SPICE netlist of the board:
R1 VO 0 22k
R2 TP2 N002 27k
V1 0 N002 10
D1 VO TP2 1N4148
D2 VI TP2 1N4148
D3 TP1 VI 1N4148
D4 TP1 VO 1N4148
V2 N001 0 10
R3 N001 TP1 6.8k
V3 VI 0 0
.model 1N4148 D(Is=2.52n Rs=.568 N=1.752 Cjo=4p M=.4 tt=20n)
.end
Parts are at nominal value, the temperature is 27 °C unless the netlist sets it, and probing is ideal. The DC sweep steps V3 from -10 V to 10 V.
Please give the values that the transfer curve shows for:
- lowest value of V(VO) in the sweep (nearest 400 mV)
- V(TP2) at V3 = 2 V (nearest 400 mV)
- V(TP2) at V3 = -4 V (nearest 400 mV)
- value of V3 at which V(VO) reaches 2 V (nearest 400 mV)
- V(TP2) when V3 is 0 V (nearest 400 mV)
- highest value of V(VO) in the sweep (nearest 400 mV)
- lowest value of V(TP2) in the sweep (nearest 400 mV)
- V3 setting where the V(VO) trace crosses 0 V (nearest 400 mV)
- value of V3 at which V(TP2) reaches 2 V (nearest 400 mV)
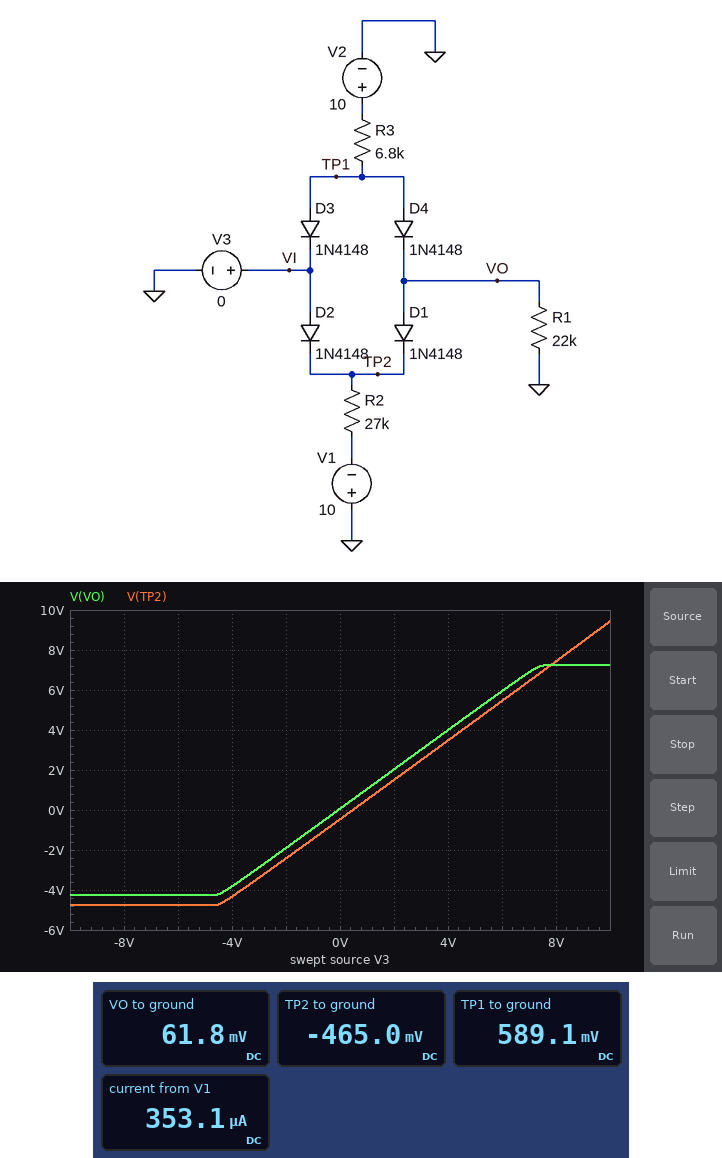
-4.4 V
1.6 V
-4.4 V
2.0 V
-400 mV
7.2 V
-4.8 V
0 V
2.4 V
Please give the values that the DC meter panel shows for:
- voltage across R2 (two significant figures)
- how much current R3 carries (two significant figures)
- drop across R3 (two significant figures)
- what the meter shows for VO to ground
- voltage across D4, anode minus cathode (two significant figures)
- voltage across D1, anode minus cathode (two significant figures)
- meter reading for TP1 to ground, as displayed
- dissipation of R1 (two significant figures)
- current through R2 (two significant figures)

9.5 V
1.4 mA
9.4 V
61.8 mV
530 mV
530 mV
589.1 mV
170 nW
350 µA
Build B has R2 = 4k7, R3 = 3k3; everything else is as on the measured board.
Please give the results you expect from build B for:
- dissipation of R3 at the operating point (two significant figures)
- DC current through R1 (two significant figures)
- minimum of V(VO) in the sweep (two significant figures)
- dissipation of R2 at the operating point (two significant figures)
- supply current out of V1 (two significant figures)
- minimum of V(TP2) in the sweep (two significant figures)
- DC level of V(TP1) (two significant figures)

27 mW
730 nA
-7.8 V
19 mW
2.0 mA
-8.3 V
610 mV
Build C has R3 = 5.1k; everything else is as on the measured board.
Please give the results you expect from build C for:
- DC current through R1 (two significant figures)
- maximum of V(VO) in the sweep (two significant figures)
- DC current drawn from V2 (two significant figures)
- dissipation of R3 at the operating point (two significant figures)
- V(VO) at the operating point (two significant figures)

3.4 µA
7.7 V
1.8 mA
17 mW
75 mV
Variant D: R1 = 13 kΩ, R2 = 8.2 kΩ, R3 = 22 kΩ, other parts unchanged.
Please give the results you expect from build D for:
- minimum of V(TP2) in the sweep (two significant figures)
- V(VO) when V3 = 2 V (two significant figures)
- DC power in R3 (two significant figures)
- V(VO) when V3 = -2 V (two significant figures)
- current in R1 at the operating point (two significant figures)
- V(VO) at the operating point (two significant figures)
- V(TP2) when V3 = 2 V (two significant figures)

-6.3 V
1.9 V
4.1 mW
-2.0 V
3.4 µA
-44 mV
1.4 V
